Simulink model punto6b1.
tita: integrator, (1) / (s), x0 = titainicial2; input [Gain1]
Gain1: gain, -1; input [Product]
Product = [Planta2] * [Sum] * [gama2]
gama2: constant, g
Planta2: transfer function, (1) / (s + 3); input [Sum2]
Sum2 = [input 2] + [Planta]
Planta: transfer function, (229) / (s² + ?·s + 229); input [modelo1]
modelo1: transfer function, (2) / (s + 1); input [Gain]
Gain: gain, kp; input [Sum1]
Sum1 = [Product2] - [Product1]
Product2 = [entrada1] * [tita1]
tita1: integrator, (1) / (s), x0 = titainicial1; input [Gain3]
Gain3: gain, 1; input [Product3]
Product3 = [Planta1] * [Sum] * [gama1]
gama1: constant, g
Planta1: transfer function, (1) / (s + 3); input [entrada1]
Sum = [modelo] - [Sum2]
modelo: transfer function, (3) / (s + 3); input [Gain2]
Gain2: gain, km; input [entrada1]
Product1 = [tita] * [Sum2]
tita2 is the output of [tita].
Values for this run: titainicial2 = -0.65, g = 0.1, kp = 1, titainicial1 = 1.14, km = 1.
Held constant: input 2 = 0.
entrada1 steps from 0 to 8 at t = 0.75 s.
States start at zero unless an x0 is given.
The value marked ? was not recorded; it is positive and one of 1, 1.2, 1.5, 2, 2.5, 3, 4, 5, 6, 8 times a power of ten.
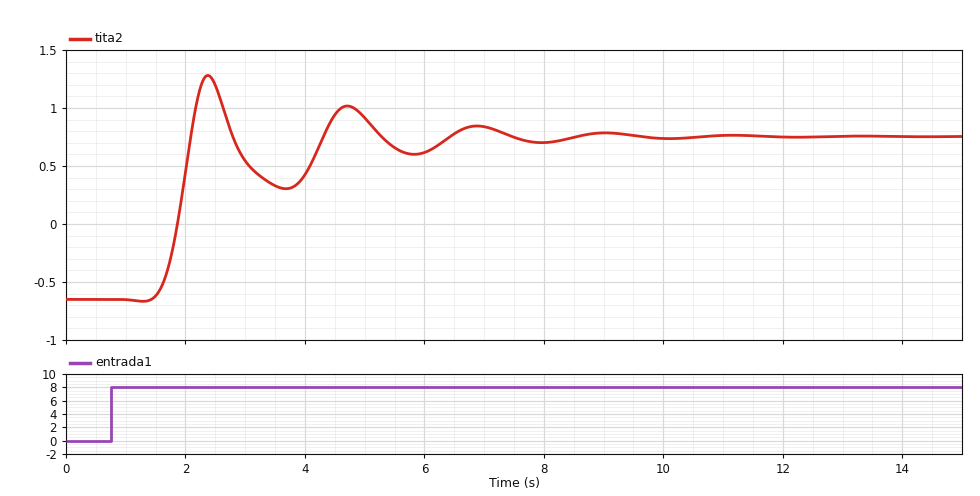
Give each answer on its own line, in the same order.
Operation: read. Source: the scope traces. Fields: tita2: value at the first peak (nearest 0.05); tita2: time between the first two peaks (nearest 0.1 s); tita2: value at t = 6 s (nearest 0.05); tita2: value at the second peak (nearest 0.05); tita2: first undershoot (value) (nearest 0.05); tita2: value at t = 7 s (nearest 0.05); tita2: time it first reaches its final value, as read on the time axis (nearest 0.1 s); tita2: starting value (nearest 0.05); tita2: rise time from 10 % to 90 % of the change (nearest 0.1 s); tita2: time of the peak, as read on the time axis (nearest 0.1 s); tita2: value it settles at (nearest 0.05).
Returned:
1.30
2.3 s
0.60
1.00
0.30
0.85
2.1 s
-0.65
0.4 s
2.4 s
0.75
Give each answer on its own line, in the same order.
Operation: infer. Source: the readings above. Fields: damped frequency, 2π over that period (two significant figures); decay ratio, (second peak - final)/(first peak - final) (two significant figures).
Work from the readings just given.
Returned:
2.7 rad/s
0.45
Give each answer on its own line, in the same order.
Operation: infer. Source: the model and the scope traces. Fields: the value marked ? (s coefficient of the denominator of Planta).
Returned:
40
